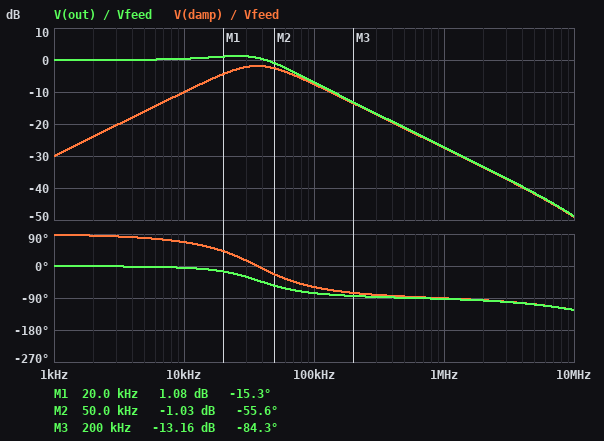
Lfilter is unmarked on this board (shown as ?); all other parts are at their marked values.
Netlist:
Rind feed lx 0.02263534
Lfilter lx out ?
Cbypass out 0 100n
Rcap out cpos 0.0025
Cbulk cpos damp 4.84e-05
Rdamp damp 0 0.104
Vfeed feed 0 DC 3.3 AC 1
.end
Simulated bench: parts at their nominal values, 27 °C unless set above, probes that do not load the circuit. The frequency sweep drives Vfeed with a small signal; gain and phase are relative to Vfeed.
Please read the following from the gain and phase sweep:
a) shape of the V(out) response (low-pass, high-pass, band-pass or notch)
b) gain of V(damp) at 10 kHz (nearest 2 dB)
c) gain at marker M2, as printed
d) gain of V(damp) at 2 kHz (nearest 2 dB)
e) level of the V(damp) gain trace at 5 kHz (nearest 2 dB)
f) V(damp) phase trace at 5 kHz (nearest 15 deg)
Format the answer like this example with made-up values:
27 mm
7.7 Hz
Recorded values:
low-pass
-10 dB
-1.03 dB
-24 dB
-16 dB
75 deg
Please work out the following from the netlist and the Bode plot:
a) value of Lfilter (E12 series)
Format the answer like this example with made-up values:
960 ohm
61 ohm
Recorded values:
390 nH
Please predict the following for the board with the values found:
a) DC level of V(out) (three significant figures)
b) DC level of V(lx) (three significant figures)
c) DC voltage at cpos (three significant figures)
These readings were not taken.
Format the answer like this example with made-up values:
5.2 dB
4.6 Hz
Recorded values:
3.30 V
3.30 V
3.30 V
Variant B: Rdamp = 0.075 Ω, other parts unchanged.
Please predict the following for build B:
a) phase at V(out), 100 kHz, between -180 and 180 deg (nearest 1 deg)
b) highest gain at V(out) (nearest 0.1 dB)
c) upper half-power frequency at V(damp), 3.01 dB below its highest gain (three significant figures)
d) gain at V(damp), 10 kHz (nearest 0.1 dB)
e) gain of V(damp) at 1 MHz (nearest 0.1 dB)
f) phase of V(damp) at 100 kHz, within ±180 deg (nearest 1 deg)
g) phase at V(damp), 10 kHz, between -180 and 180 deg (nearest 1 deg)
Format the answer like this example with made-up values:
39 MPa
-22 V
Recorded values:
-88 deg
2.0 dB
62.3 kHz
-12.6 dB
-30.3 dB
-65 deg
72 deg
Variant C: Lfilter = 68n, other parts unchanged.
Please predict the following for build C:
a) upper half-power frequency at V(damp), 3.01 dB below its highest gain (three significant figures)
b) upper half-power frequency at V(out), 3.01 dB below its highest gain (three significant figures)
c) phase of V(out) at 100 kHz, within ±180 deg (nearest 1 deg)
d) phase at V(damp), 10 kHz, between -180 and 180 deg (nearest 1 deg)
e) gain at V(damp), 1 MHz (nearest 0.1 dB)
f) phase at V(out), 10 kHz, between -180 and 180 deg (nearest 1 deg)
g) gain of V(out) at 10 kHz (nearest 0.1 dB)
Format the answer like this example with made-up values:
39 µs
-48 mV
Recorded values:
330 kHz
226 kHz
-22 deg
68 deg
-12.5 dB
-4 deg
-0.1 dB
